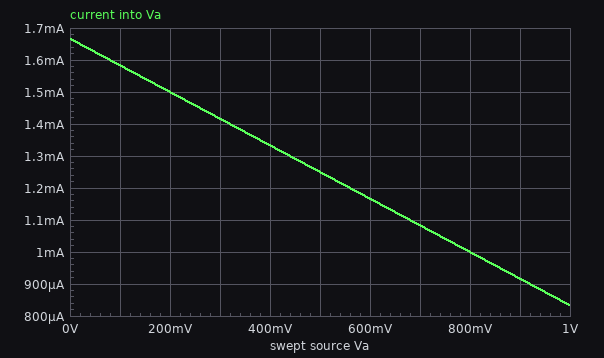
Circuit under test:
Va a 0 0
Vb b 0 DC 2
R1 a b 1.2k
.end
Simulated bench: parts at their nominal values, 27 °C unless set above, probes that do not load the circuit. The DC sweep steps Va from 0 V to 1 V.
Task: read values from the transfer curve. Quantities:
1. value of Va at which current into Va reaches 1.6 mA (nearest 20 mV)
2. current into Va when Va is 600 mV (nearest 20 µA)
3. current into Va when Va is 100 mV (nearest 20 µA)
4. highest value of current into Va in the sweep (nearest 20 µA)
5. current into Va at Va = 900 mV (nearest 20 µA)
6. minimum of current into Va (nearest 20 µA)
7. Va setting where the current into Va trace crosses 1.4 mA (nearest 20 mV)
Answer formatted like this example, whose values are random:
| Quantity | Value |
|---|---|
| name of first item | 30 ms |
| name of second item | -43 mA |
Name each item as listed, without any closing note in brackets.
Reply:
| Quantity | Value |
|---|---|
| value of Va at which current into Va reaches 1.6 mA | 80 mV |
| current into Va when Va is 600 mV | 1.16 mA |
| current into Va when Va is 100 mV | 1.58 mA |
| highest value of current into Va in the sweep | 1.66 mA |
| current into Va at Va = 900 mV | 920 µA |
| minimum of current into Va | 840 µA |
| Va setting where the current into Va trace crosses 1.4 mA | 320 mV |
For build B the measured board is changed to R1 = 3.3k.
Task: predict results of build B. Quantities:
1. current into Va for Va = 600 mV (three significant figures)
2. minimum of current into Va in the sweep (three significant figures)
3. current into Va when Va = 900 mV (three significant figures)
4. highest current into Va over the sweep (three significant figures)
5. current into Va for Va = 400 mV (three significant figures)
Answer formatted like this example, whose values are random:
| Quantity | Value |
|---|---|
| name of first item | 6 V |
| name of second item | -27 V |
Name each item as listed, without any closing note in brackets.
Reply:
| Quantity | Value |
|---|---|
| current into Va for Va = 600 mV | 424 µA |
| minimum of current into Va in the sweep | 303 µA |
| current into Va when Va = 900 mV | 333 µA |
| highest current into Va over the sweep | 606 µA |
| current into Va for Va = 400 mV | 485 µA |
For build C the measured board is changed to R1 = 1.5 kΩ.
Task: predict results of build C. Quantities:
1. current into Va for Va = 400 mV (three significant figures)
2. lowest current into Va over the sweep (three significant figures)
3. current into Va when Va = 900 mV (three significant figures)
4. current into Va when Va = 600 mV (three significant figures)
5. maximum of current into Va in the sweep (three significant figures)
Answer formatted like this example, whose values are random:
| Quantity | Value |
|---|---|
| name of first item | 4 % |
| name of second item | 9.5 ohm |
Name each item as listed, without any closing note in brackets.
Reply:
| Quantity | Value |
|---|---|
| current into Va for Va = 400 mV | 1.07 mA |
| lowest current into Va over the sweep | 667 µA |
| current into Va when Va = 900 mV | 733 µA |
| current into Va when Va = 600 mV | 933 µA |
| maximum of current into Va in the sweep | 1.33 mA |
